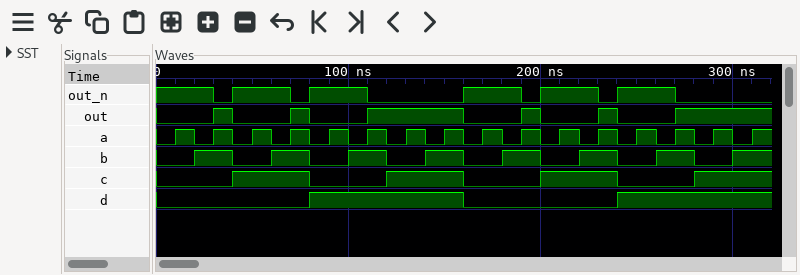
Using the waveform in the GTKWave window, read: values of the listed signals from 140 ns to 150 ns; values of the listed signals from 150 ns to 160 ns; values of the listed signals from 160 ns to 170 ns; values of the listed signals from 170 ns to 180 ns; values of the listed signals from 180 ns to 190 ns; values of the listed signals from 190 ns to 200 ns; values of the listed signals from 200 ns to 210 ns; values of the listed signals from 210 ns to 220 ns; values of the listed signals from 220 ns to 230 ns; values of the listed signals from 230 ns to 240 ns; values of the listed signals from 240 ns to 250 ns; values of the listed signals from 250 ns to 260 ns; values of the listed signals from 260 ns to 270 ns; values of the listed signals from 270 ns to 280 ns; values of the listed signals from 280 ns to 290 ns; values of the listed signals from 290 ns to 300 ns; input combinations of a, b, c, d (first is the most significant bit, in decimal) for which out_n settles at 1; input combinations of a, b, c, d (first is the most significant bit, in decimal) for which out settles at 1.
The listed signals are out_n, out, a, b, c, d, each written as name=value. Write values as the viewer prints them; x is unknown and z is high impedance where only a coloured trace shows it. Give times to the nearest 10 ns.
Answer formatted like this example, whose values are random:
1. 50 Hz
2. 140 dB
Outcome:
1. out_n=0, out=1, a=0, b=1, c=1, d=1
2. out_n=0, out=1, a=1, b=1, c=1, d=1
3. out_n=1, out=0, a=0, b=0, c=0, d=0
4. out_n=1, out=0, a=1, b=0, c=0, d=0
5. out_n=1, out=0, a=0, b=1, c=0, d=0
6. out_n=0, out=1, a=1, b=1, c=0, d=0
7. out_n=1, out=0, a=0, b=0, c=1, d=0
8. out_n=1, out=0, a=1, b=0, c=1, d=0
9. out_n=1, out=0, a=0, b=1, c=1, d=0
10. out_n=0, out=1, a=1, b=1, c=1, d=0
11. out_n=1, out=0, a=0, b=0, c=0, d=1
12. out_n=1, out=0, a=1, b=0, c=0, d=1
13. out_n=1, out=0, a=0, b=1, c=0, d=1
14. out_n=0, out=1, a=1, b=1, c=0, d=1
15. out_n=0, out=1, a=0, b=0, c=1, d=1
16. out_n=0, out=1, a=1, b=0, c=1, d=1
17. 0, 1, 2, 4, 5, 6, 8, 9, 10
18. 3, 7, 11, 12, 13, 14, 15
